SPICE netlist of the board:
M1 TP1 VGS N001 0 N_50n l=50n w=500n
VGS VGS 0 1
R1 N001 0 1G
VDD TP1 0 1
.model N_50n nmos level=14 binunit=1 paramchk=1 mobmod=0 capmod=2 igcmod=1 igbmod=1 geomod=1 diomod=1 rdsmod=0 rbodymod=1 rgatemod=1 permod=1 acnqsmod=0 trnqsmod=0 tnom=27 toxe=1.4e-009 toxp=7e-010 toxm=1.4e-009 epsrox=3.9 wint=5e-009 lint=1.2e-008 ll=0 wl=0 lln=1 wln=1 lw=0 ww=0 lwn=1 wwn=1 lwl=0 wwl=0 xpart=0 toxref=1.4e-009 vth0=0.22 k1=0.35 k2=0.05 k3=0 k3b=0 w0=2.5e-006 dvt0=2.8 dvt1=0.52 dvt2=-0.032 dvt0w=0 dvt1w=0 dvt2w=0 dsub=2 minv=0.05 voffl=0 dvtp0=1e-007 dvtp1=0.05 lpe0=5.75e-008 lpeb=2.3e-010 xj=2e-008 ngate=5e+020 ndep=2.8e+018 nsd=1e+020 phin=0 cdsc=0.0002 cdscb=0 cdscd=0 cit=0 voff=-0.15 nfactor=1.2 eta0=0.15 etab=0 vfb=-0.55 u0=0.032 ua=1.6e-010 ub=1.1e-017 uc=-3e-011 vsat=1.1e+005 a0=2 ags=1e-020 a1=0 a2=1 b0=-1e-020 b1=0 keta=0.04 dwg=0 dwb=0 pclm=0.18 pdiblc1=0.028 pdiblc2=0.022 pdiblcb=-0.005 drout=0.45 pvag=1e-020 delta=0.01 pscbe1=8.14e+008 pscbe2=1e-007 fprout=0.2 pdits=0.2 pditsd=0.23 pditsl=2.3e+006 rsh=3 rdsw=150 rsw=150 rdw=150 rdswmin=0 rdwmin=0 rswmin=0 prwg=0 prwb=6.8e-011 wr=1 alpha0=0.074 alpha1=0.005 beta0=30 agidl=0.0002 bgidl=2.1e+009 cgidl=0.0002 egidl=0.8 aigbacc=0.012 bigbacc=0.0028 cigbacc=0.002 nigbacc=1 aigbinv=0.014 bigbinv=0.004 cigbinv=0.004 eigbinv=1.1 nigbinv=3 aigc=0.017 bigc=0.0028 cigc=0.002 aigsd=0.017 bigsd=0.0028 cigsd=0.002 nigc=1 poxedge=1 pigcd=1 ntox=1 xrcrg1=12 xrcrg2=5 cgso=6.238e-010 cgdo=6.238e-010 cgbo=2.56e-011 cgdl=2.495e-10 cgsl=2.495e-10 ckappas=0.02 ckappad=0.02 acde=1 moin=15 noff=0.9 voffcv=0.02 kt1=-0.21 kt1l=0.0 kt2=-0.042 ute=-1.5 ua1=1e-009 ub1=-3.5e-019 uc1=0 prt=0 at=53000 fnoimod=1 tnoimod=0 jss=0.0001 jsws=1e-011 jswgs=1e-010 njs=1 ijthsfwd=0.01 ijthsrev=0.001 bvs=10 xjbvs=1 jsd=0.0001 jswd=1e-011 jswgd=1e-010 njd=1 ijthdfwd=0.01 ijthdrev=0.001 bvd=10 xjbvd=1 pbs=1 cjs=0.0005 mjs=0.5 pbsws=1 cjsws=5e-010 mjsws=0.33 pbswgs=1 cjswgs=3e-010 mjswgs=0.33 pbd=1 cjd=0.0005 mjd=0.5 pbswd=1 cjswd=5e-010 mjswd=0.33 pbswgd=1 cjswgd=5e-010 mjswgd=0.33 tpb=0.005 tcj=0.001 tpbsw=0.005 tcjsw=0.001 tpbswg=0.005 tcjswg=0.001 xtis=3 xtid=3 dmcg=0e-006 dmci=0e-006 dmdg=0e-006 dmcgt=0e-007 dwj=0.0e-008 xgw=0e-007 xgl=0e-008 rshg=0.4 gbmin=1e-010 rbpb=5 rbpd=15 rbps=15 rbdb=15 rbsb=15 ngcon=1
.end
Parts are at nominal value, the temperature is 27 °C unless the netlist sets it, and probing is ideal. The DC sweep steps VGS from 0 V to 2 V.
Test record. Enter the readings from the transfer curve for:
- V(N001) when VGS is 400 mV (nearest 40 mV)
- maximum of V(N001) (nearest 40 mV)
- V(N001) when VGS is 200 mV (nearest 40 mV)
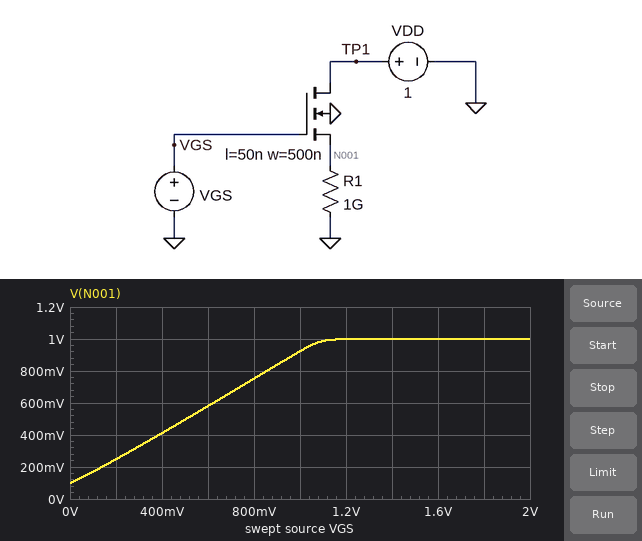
400 mV
1.00 V
240 mV
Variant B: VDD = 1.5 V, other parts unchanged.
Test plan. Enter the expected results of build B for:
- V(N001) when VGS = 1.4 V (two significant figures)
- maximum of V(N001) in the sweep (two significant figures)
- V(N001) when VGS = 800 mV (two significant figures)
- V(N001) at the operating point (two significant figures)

1.3 V
1.5 V
770 mV
940 mV
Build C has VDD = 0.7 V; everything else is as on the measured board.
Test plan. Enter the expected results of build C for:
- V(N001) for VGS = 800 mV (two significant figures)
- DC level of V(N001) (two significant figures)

690 mV
700 mV
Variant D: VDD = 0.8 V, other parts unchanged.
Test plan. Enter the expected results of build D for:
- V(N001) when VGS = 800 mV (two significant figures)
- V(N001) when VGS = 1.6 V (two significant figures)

740 mV
800 mV
